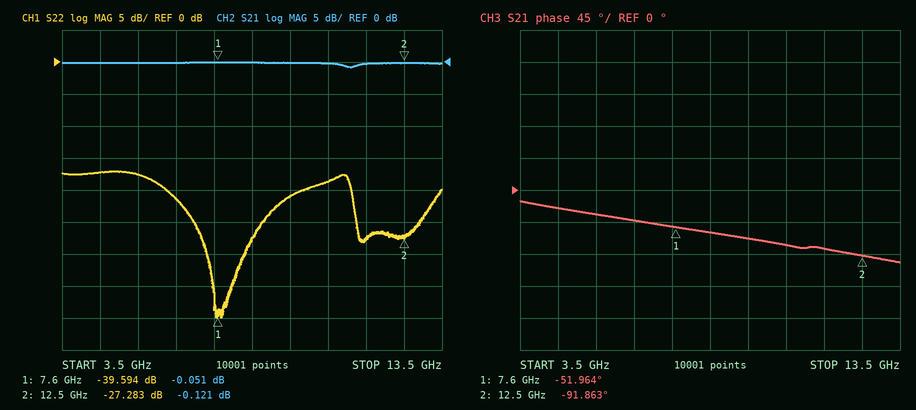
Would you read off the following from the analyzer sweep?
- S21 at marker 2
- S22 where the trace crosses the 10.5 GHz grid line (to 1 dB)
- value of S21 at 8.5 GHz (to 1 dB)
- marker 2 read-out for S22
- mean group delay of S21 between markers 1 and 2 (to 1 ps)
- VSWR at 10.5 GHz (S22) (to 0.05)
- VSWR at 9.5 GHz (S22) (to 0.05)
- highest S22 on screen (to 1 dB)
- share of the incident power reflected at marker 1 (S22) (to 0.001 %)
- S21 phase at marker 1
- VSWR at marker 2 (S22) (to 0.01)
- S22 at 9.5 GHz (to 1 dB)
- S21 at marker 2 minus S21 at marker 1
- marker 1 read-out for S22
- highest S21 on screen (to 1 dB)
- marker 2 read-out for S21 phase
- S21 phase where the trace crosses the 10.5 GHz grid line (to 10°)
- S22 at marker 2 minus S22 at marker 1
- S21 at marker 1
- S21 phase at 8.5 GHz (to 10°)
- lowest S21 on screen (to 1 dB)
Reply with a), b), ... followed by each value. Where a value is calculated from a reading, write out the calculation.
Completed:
a) -0.121 dB
b) -19 dB
c) 0 dB
d) -27.283 dB
e) −(-91.863° − (-51.964°))/(360° × 4.9 GHz) ≈ 23 ps
f) |Γ| = 10^(-19/20) = 0.1122; VSWR = (1 + 0.1122)/(1 − 0.1122) ≈ 1.25
g) |Γ| = 10^(-21/20) = 0.0891; VSWR = (1 + 0.0891)/(1 − 0.0891) ≈ 1.20
h) -17 dB
i) 10^(-39.594/10) ≈ 0.011 %
j) -51.964°
k) (1 + 0.0432)/(1 − 0.0432) ≈ 1.09
l) -21 dB
m) -0.121 − (-0.051) = -0.070 dB
n) -39.594 dB
o) 0 dB
p) -91.863°
q) -80°
r) -27.283 − (-39.594) = 12.311 dB
s) -0.051 dB
t) -60°
u) -1 dB
